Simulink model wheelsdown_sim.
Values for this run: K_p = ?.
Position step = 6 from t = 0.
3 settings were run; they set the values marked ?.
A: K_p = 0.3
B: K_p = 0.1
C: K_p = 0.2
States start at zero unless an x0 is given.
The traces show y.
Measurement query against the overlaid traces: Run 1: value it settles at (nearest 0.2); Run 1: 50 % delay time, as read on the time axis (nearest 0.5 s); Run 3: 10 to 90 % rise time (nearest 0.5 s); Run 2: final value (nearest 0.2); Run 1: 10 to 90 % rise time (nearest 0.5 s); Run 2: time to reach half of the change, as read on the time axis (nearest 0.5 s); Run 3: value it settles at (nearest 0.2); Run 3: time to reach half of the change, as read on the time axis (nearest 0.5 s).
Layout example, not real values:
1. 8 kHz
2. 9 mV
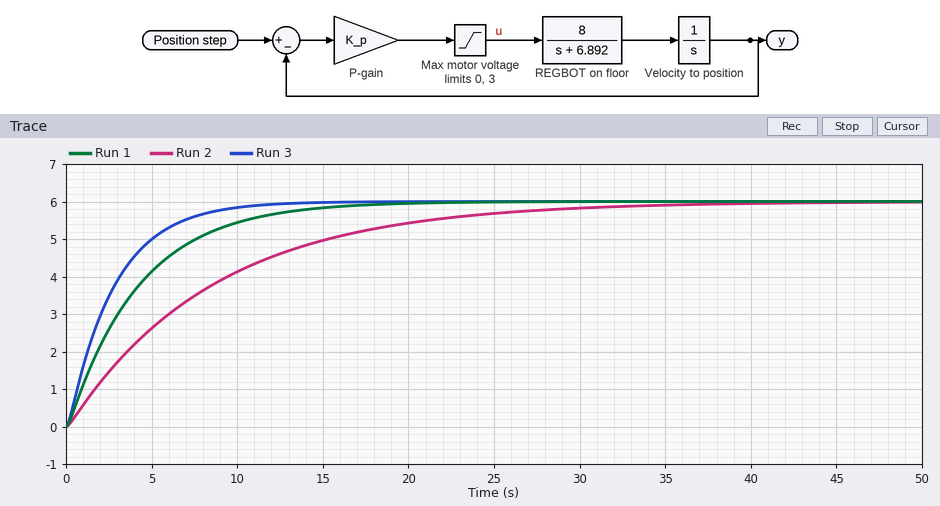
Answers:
1. 6.0
2. 3.0 s
3. 6.0 s
4. 6.0
5. 9.0 s
6. 6.0 s
7. 6.0
8. 2.0 s
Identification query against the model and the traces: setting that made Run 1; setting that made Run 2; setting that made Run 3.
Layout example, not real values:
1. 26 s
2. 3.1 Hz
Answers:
1. C
2. B
3. A
